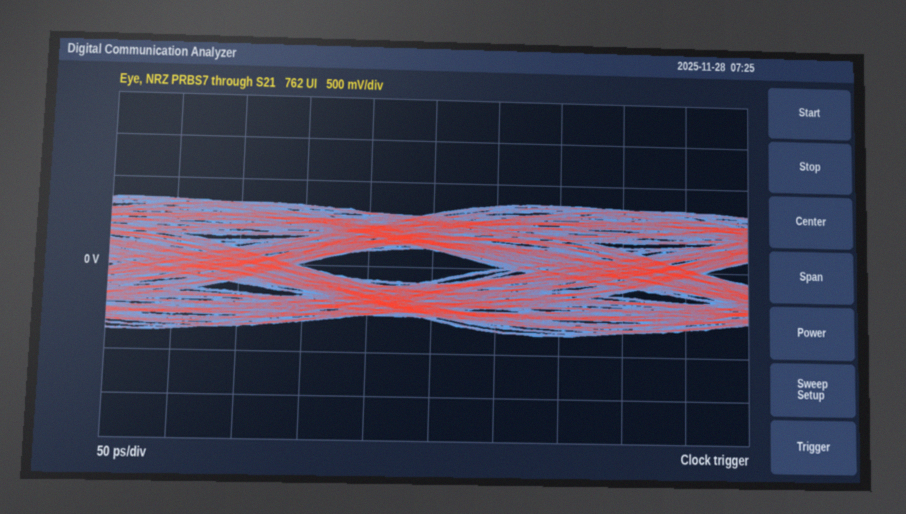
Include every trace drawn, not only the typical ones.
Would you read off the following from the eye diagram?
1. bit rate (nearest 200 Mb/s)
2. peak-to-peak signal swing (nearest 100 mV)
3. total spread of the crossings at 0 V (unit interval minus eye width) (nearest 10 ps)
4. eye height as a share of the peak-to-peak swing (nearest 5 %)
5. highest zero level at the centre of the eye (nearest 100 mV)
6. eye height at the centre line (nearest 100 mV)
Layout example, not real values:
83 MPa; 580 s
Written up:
3.2 Gb/s; 1.5 V; 160 ps; 25 %; -200 mV; 400 mV
